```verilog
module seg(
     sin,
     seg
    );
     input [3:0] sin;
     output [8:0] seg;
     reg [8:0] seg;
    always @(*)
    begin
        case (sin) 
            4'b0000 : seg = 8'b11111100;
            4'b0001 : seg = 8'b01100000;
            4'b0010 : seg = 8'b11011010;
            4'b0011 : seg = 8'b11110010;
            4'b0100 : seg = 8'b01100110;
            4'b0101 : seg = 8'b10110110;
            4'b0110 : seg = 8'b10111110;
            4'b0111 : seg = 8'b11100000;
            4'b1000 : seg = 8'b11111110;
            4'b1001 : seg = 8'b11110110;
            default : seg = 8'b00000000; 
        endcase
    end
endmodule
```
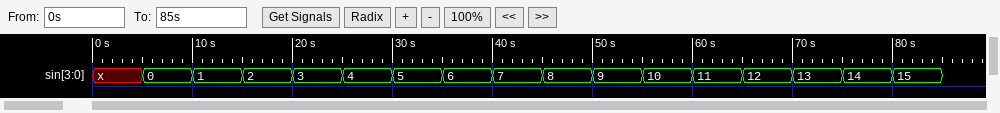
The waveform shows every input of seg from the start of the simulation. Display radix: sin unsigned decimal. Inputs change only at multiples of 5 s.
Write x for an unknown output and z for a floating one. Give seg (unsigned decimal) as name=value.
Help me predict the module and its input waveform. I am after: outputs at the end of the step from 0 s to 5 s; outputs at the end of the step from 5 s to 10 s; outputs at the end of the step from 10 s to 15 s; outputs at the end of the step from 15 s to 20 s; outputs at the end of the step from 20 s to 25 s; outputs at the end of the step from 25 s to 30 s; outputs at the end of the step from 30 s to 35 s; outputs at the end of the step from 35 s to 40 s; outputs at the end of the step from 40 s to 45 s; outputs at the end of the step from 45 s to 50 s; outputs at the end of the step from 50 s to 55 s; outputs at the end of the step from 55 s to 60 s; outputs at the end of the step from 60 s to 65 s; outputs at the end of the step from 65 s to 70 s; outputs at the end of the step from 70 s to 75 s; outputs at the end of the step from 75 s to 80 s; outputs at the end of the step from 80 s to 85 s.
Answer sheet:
seg=x
seg=252
seg=96
seg=218
seg=242
seg=102
seg=182
seg=190
seg=224
seg=254
seg=246
seg=0
seg=0
seg=0
seg=0
seg=0
seg=0
